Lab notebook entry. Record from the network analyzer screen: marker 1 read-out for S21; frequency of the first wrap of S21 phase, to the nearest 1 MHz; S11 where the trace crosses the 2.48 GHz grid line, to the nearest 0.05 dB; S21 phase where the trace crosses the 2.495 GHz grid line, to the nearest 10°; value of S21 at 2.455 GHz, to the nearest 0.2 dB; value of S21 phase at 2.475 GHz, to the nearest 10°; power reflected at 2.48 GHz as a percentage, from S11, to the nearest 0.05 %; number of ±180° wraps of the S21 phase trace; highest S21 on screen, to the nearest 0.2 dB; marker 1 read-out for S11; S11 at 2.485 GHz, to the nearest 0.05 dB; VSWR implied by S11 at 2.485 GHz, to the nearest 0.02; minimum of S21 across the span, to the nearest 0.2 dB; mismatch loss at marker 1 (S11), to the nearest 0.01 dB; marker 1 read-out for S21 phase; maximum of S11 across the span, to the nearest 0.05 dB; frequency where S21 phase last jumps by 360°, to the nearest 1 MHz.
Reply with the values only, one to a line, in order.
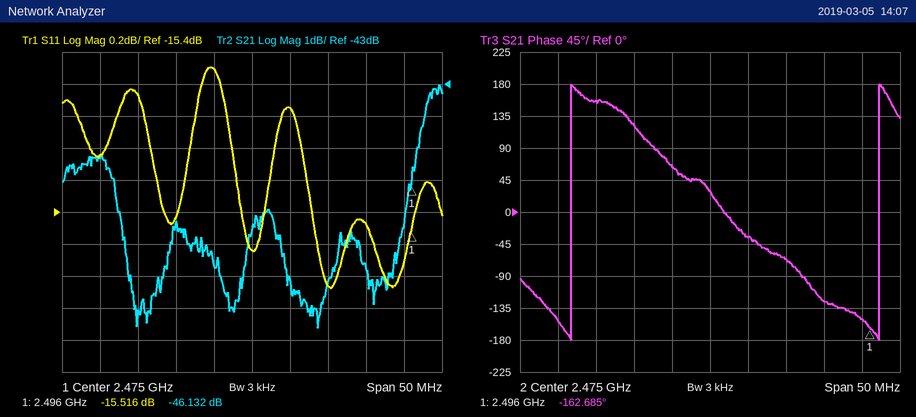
-46.132 dB
2.457 GHz
-14.75 dB
-150°
-45.4 dB
30°
3.35 %
2
-43.0 dB
-15.516 dB
-15.85 dB
1.38
-50.6 dB
0.12 dB
-162.685°
-14.50 dB
2.497 GHz
